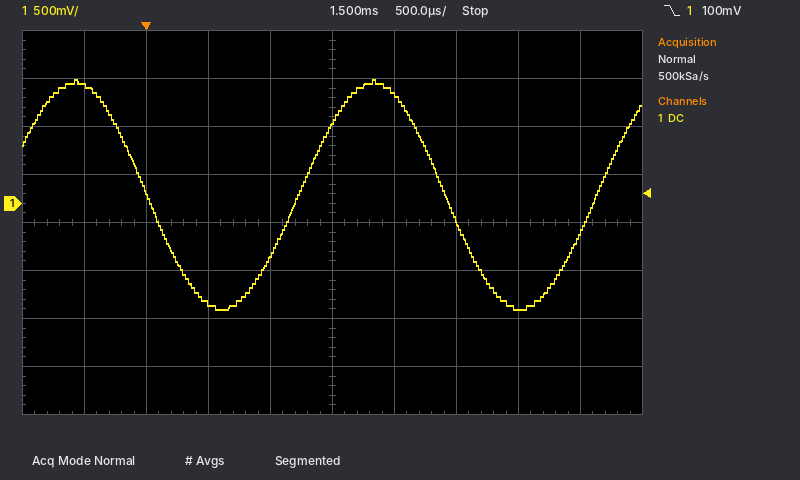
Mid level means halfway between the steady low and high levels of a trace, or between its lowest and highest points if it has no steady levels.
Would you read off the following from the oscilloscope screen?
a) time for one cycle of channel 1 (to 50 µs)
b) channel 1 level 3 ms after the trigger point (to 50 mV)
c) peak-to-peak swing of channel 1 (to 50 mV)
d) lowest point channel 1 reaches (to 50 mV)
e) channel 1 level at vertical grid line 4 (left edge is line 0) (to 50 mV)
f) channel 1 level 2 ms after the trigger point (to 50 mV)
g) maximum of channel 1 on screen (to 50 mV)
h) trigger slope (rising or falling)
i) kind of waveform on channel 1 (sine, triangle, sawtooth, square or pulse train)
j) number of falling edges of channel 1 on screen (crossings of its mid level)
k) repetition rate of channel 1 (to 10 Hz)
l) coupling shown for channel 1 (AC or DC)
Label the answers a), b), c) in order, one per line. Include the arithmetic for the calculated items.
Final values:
a) 2.40 ms
b) -1.10 V
c) 1.30 V − (-1.10 V) = 2.40 V
d) -1.10 V
e) -550 mV
f) 1.15 V
g) 1.30 V
h) falling
i) sine
j) 2
k) 1 / 2.40 ms ≈ 417 Hz, so 420 Hz to the nearest 10 Hz
l) DC
